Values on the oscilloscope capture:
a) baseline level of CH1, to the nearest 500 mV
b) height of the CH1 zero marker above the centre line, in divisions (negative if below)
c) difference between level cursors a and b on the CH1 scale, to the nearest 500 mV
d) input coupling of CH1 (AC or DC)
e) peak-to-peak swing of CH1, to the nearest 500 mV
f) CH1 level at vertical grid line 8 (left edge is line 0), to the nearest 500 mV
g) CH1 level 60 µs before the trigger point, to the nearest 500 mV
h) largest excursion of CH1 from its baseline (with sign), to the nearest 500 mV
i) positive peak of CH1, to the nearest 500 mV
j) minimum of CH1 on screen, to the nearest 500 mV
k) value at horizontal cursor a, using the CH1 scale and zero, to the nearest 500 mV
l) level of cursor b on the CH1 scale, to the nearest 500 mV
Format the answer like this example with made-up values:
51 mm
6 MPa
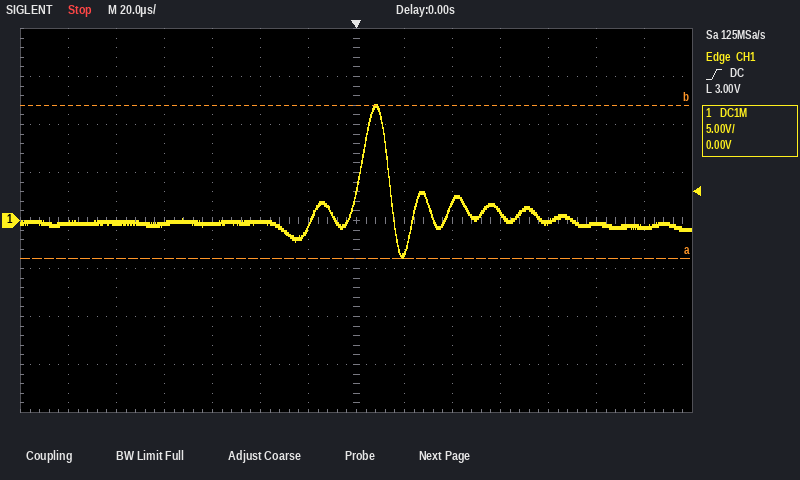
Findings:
-500 mV
0.0 div
16.0 V
DC
16.0 V
-3.5 V
-500 mV
+12.5 V
12.0 V
-4.0 V
-4.0 V
12.0 V
